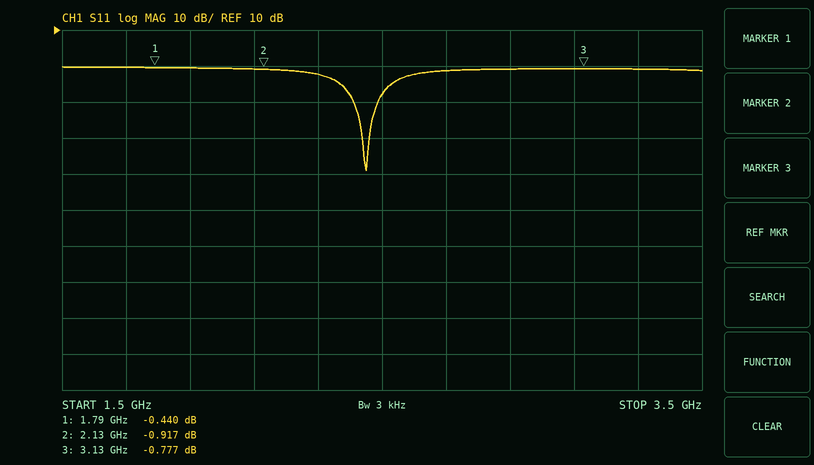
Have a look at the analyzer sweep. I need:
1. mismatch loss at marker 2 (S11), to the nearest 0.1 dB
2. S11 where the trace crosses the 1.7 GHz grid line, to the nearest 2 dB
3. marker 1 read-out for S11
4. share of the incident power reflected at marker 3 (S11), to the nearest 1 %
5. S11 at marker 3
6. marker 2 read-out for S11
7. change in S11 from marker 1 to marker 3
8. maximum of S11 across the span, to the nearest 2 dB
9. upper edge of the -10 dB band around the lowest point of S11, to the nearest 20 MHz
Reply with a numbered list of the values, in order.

1. 7.2 dB
2. 0 dB
3. -0.440 dB
4. 84 %
5. -0.777 dB
6. -0.917 dB
7. -0.337 dB
8. 0 dB
9. 2.48 GHz
